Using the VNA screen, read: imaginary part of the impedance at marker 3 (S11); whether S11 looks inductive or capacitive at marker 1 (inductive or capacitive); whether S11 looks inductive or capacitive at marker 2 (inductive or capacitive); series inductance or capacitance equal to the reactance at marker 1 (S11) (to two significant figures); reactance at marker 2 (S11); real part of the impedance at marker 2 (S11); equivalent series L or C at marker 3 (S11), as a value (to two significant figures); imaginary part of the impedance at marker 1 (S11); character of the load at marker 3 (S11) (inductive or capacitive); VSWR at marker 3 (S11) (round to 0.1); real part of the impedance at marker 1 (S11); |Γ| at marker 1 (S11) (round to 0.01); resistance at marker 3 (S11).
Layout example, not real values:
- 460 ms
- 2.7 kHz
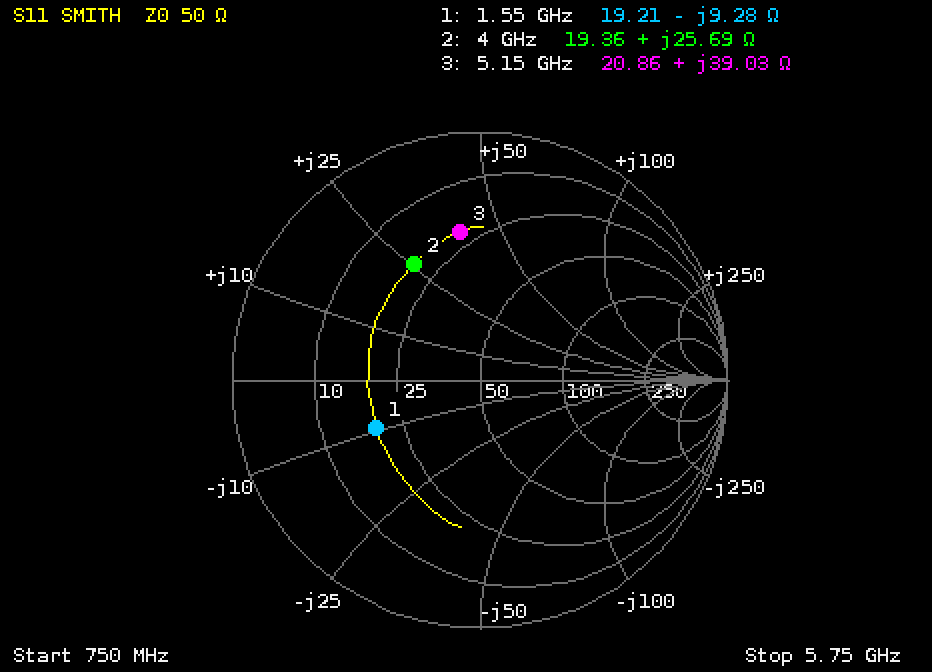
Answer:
- +39.03 Ω
- capacitive
- inductive
- 11 pF
- +25.69 Ω
- 19.36 Ω
- 1.2 nH
- -9.28 Ω
- inductive
- 4.0
- 19.21 Ω
- 0.46
- 20.86 Ω
